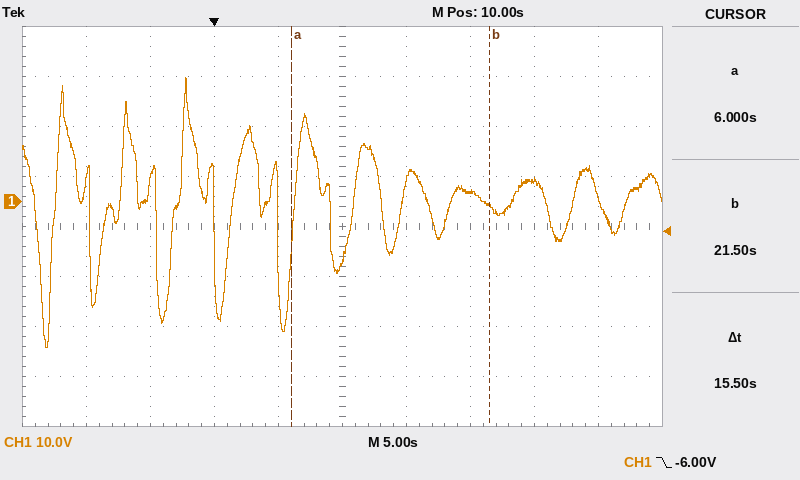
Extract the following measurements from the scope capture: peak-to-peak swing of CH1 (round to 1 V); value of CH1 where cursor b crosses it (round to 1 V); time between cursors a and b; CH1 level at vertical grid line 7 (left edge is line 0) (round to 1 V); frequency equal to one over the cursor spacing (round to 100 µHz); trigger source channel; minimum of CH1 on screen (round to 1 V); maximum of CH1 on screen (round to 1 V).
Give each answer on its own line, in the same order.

54 V
-1 V
15.5 s
2 V
64.5 mHz
CH1
-29 V
25 V
